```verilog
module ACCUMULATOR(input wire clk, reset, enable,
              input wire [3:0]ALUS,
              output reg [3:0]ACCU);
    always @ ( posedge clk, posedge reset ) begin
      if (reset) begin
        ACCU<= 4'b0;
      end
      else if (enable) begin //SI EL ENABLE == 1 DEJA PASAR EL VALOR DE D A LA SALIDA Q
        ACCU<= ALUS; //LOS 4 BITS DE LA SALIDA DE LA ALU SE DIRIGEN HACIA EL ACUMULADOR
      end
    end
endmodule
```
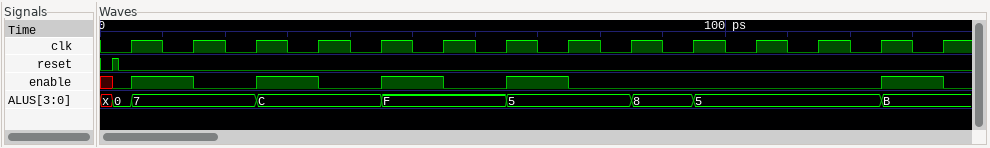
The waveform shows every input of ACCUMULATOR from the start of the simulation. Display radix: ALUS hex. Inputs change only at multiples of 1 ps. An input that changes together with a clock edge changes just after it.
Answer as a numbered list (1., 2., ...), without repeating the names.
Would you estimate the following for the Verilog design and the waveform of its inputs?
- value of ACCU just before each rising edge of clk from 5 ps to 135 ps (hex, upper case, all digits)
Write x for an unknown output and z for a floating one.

1. 0, 0, 7, 7, C, C, F, F, 5, 5, 5, 5, 5, 5
